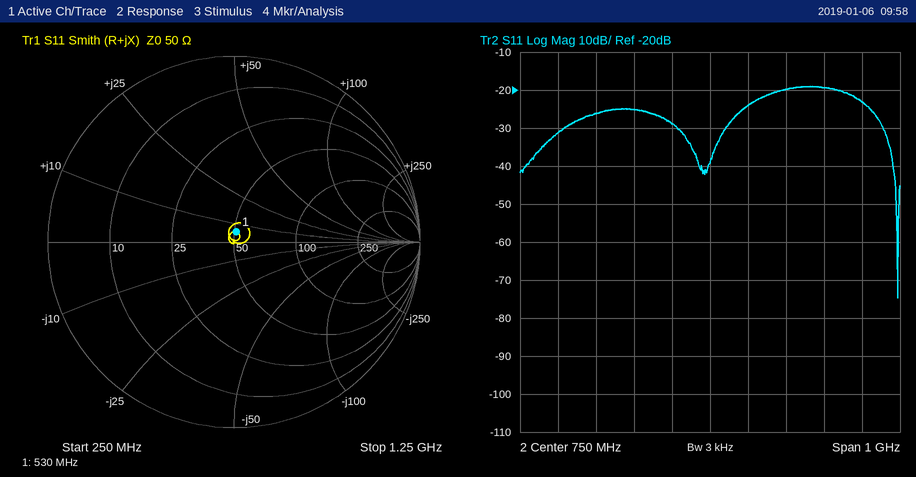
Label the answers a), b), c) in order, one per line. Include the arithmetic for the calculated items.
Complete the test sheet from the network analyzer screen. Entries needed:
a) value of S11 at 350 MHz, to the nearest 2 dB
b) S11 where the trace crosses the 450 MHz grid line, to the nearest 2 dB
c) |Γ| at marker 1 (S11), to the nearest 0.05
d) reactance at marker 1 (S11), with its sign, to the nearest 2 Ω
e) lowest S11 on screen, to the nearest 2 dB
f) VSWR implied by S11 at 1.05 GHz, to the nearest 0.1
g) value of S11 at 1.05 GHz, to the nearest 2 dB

a) -32 dB
b) -26 dB
c) 0.05
d) +6 Ω
e) -74 dB
f) |Γ| = 10^(-20/20) = 0.1000; VSWR = (1 + 0.1000)/(1 − 0.1000) ≈ 1.2
g) -20 dB
